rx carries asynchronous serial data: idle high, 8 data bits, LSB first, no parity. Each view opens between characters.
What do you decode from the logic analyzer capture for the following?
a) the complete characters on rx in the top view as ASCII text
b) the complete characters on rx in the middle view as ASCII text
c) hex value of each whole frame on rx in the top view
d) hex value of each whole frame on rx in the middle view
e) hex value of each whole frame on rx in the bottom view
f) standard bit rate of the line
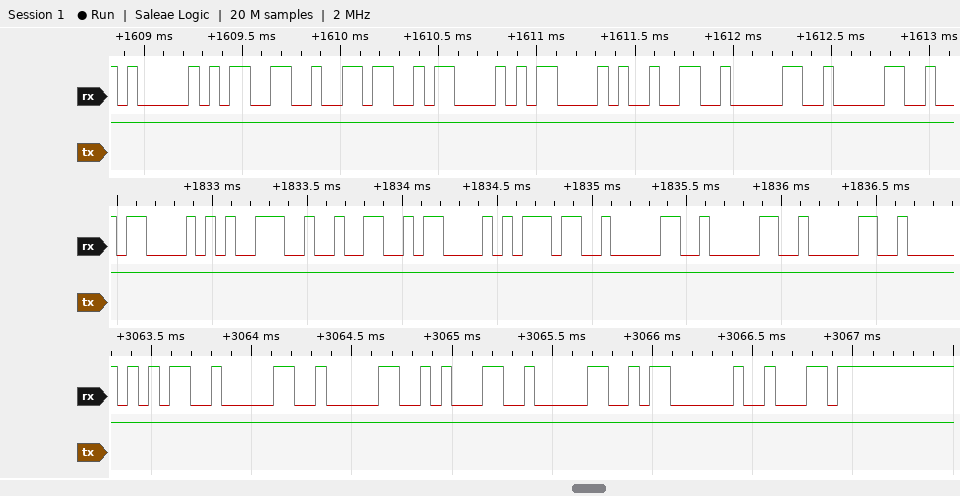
"A36CC200"
"C92C7000"
41, 33, 36, 43, 43, 32, 30, 30
43, 39, 32, 43, 37, 30, 30, 30
35, 30, 30, 31, 30, 03, 62
19200 baud
